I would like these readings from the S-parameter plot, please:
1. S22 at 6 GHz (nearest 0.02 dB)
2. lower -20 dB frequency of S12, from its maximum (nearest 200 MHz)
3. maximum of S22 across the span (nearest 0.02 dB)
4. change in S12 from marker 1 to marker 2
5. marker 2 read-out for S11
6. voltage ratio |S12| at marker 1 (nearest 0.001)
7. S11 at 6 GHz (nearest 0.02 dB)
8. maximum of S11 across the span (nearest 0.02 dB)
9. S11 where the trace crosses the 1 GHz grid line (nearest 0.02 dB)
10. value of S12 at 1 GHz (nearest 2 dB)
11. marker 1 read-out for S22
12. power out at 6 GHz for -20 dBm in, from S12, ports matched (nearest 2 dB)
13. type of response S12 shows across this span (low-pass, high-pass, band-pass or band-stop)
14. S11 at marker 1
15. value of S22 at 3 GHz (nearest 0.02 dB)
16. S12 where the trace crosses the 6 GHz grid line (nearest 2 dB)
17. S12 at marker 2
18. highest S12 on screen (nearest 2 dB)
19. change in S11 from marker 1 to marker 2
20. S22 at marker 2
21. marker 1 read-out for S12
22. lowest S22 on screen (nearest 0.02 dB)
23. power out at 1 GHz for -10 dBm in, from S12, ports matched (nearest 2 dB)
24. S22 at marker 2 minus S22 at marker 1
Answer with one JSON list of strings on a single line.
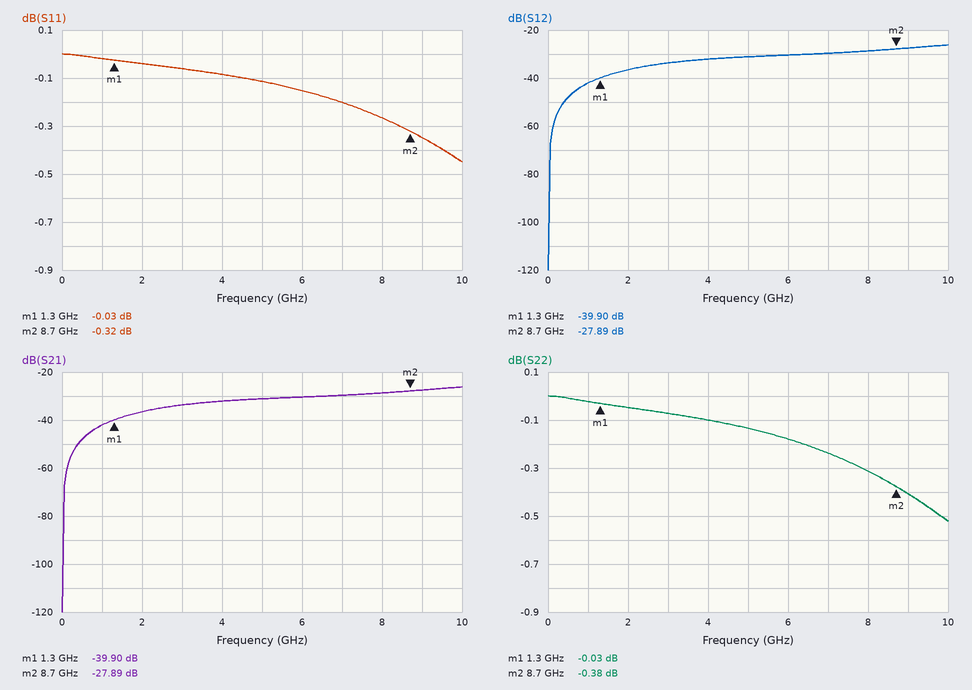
["-0.18 dB", "600 MHz", "0.00 dB", "12.01 dB", "-0.32 dB", "0.010", "-0.16 dB", "0.00 dB", "-0.02 dB", "-42 dB", "-0.03 dB", "-50 dBm", "high-pass", "-0.03 dB", "-0.08 dB", "-30 dB", "-27.89 dB", "-26 dB", "-0.29 dB", "-0.38 dB", "-39.90 dB", "-0.52 dB", "-52 dBm", "-0.35 dB"]
